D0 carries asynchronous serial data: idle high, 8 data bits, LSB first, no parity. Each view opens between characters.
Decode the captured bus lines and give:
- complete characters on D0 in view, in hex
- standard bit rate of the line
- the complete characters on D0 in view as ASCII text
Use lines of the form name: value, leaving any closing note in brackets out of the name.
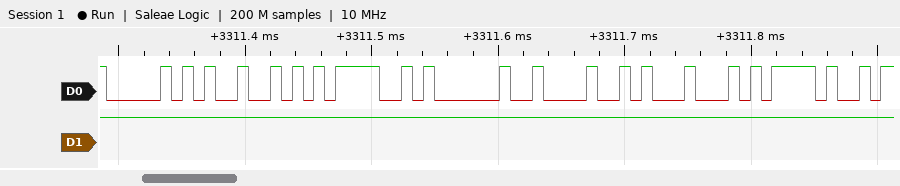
complete characters on D0 in view, in hex: 50, 52, 4F, 20, 48, 44, 2F
standard bit rate of the line: 115200 baud
the complete characters on D0 in view as ASCII text: "PRO HD/"
